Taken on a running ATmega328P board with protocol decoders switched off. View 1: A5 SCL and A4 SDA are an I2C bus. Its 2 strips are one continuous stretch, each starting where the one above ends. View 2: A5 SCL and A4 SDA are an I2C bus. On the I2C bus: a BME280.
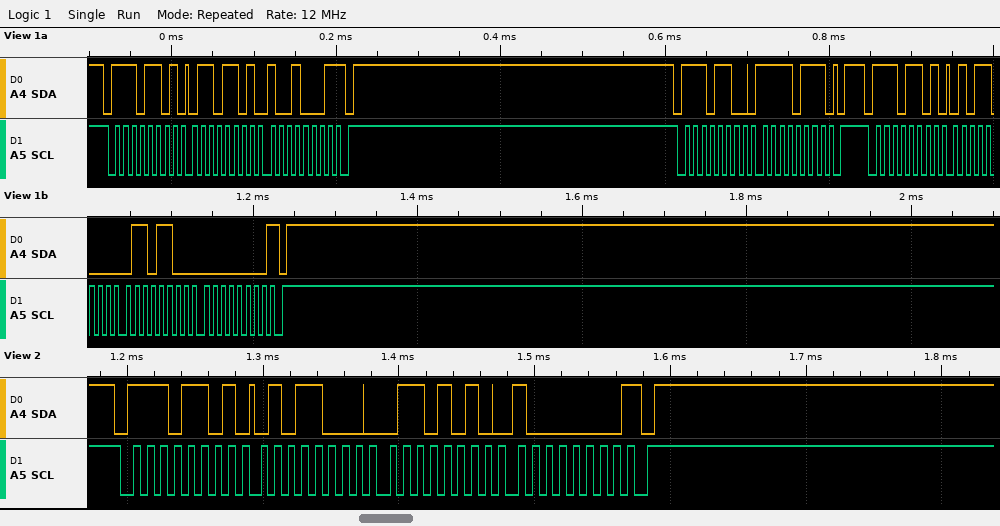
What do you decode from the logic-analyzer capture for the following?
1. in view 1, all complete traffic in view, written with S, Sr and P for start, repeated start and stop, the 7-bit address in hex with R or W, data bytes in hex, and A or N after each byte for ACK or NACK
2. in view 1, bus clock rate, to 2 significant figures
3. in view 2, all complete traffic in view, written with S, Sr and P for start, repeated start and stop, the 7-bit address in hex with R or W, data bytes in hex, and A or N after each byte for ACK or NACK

S 76R A 6D A 91 N P S 76W A F7 A P S 76R A 58 A 6C A 00 N P
100 kHz
S 76R A 58 A 6A A 80 N P
